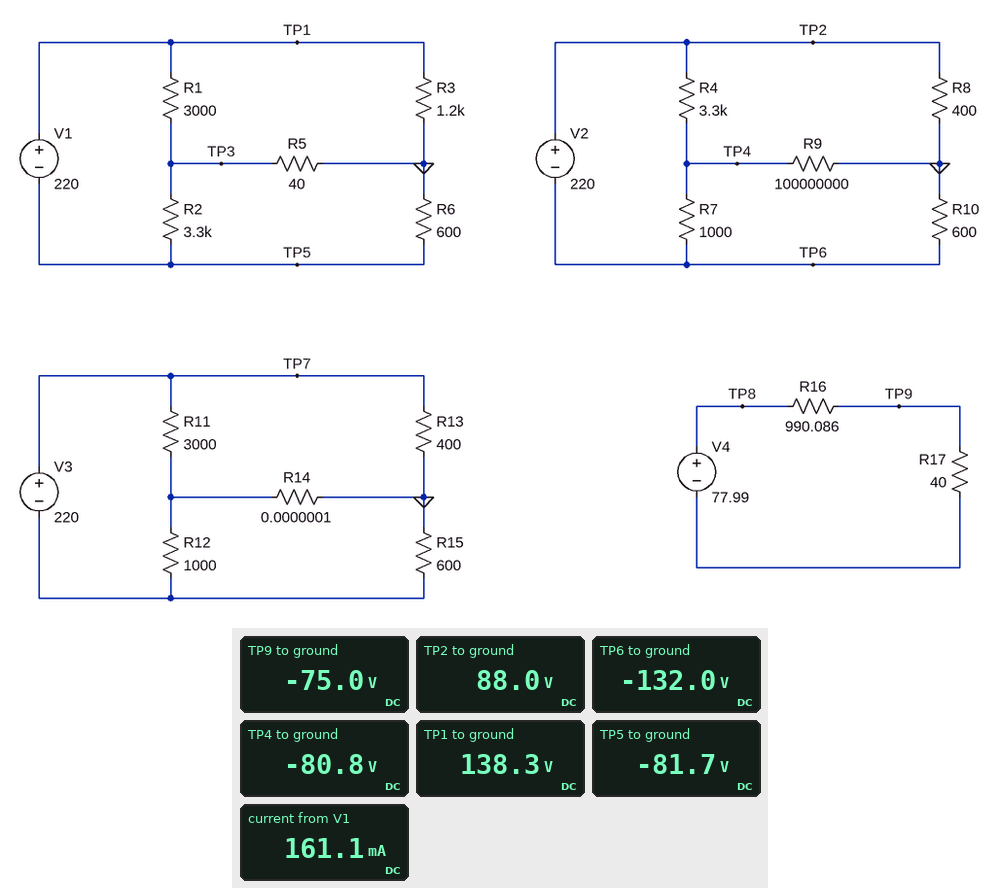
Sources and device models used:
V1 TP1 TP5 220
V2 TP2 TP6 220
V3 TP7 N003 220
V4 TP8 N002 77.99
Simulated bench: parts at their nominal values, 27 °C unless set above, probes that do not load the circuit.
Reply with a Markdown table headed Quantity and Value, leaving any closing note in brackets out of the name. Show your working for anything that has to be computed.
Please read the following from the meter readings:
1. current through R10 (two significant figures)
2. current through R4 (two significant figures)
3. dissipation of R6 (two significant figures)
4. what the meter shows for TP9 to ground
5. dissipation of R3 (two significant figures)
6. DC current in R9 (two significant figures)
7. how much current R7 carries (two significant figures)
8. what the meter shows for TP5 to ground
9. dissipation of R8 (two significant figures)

| Quantity | Value |
|---|---|
| current through R10 | (0 V - (-132 V)) / 600 Ω = 220 mA |
| current through R4 | (88 V - (-80.8 V)) / 3.3 kΩ = 51 mA |
| dissipation of R6 | (0 V - (-81.7 V))^2 / 600 Ω = 11 W |
| what the meter shows for TP9 to ground | -75.0 V |
| dissipation of R3 | (138.3 V)^2 / 1.2 kΩ = 16 W |
| DC current in R9 | (0 V - (-80.8 V)) / 100 MΩ = 810 nA |
| how much current R7 carries | (-80.8 V - (-132 V)) / 1 kΩ = 51 mA |
| what the meter shows for TP5 to ground | -81.7 V |
| dissipation of R8 | (88 V)^2 / 400 Ω = 19 W |
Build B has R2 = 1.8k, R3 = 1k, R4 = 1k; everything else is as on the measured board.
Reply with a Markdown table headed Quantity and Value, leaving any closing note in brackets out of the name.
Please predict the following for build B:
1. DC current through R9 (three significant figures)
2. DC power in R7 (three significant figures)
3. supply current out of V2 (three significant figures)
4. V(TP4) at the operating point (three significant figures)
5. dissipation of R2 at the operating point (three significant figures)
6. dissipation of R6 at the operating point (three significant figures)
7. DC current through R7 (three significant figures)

| Quantity | Value |
|---|---|
| DC current through R9 | 220 nA |
| DC power in R7 | 12.1 W |
| supply current out of V2 | 330 mA |
| V(TP4) at the operating point | -22.0 V |
| dissipation of R2 at the operating point | 3.78 W |
| dissipation of R6 at the operating point | 11.3 W |
| DC current through R7 | 110 mA |
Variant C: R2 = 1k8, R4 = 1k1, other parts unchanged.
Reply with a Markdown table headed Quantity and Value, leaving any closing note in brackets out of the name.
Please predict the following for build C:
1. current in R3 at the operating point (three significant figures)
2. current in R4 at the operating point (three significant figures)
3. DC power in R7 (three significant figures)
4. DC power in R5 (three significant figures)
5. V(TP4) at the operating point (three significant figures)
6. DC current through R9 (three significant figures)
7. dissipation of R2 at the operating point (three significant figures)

| Quantity | Value |
|---|---|
| current in R3 at the operating point | 120 mA |
| current in R4 at the operating point | 105 mA |
| DC power in R7 | 11.0 W |
| DC power in R5 | 1.37 mW |
| V(TP4) at the operating point | -27.2 V |
| DC current through R9 | 272 nA |
| dissipation of R2 at the operating point | 3.20 W |
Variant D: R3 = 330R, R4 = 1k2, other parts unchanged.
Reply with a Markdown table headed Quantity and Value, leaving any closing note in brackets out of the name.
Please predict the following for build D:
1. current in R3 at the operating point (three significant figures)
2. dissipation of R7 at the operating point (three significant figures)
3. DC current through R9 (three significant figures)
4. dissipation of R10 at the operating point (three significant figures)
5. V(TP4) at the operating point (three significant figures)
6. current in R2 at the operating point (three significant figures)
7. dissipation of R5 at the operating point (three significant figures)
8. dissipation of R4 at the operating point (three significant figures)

| Quantity | Value |
|---|---|
| current in R3 at the operating point | 246 mA |
| dissipation of R7 at the operating point | 10.0 W |
| DC current through R9 | 320 nA |
| dissipation of R10 at the operating point | 29.0 W |
| V(TP4) at the operating point | -32.0 V |
| current in R2 at the operating point | 41.9 mA |
| dissipation of R5 at the operating point | 8.57 mW |
| dissipation of R4 at the operating point | 12.0 W |
